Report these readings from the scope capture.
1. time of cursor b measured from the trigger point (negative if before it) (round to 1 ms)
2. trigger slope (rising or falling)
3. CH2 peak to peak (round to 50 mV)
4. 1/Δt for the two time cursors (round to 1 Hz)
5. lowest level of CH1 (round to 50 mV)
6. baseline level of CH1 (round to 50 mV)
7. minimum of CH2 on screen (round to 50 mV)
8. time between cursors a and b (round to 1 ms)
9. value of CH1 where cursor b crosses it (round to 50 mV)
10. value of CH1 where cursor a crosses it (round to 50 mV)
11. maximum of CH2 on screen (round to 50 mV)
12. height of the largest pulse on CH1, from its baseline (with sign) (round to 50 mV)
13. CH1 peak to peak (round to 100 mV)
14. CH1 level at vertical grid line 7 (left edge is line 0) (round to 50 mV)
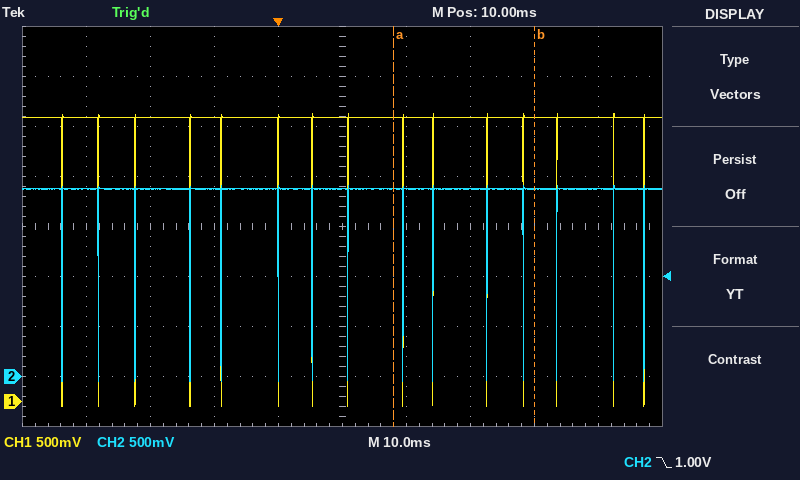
+40 ms
falling
1.95 V
45 Hz
-50 mV
2.85 V
-50 mV
22 ms
2.85 V
2.85 V
1.90 V
-2.90 V
2.90 V
2.85 V
